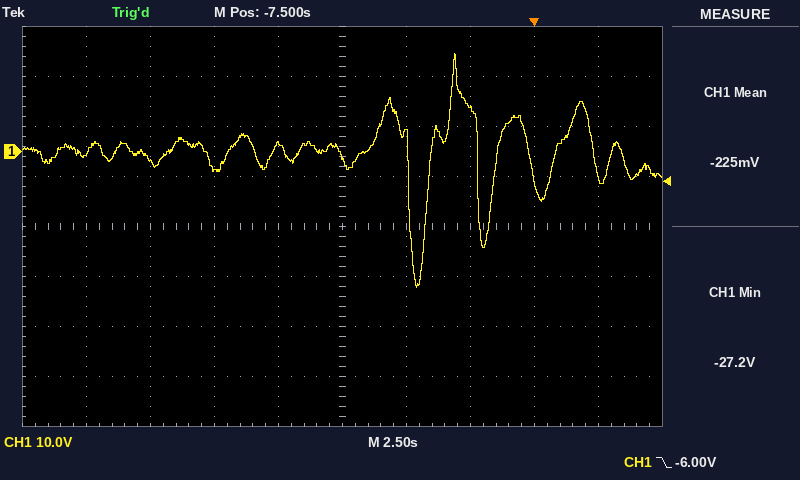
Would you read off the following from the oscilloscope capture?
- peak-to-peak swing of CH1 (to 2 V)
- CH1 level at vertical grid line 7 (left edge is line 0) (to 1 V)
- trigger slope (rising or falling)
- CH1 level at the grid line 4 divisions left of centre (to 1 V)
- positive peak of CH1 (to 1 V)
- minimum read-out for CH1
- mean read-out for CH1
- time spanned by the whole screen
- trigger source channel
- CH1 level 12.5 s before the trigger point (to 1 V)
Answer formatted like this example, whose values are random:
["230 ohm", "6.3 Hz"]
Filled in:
["46 V", "9 V", "falling", "0 V", "20 V", "-27.2 V", "-225 mV", "25 s", "CH1", "-3 V"]
